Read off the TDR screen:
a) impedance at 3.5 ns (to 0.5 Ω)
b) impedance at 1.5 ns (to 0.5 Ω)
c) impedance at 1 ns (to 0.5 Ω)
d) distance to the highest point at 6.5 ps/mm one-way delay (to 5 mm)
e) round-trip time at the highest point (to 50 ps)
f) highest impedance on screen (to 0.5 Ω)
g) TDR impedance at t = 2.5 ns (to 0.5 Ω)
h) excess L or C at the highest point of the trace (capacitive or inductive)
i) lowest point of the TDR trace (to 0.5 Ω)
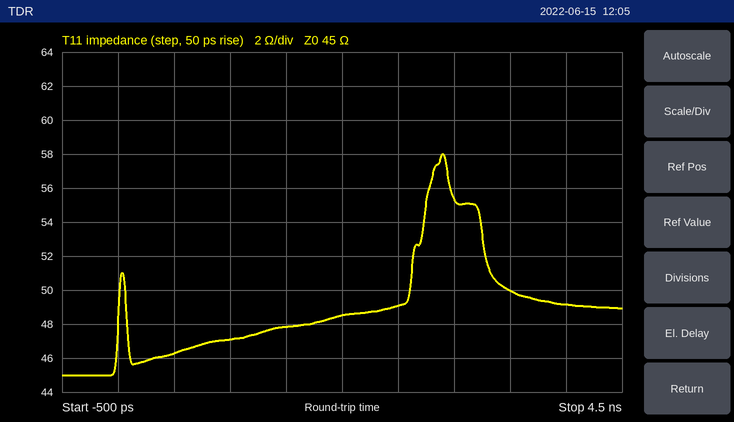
50.0 Ω
48.0 Ω
47.0 Ω
225 mm
2.90 ns
58.0 Ω
49.0 Ω
inductive
45.0 Ω
